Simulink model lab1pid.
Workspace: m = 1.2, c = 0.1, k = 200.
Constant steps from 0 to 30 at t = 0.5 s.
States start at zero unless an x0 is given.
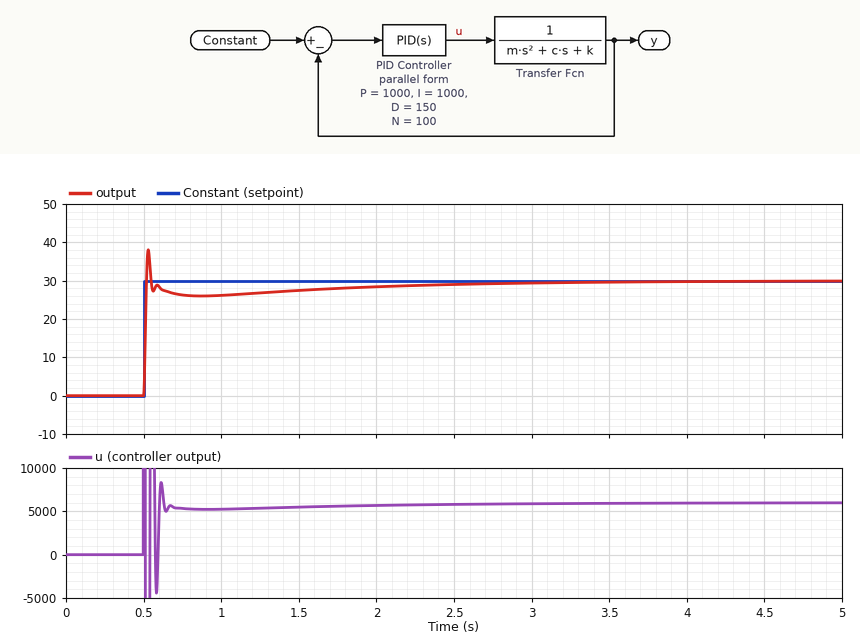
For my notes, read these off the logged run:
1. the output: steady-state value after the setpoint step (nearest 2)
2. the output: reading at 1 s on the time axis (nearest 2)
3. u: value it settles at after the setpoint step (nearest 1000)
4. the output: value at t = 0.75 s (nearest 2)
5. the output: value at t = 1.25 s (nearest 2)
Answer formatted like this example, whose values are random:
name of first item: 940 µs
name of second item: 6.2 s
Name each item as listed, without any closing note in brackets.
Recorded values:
the output: steady-state value after the setpoint step: 30
the output: reading at 1 s on the time axis: 26
u: value it settles at after the setpoint step: 6000
the output: value at t = 0.75 s: 26
the output: value at t = 1.25 s: 26
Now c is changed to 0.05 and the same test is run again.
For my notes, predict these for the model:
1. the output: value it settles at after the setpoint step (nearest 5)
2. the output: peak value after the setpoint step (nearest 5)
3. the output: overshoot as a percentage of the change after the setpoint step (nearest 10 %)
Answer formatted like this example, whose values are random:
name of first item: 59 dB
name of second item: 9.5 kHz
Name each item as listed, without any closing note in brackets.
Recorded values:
the output: value it settles at after the setpoint step: 30
the output: peak value after the setpoint step: 40
the output: overshoot as a percentage of the change after the setpoint step: 30 %
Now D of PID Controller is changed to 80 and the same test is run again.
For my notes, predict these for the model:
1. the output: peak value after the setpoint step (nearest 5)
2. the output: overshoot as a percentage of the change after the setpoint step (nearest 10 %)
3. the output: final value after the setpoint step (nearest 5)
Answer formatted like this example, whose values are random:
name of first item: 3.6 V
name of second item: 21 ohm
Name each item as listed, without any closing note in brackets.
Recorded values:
the output: peak value after the setpoint step: 35
the output: overshoot as a percentage of the change after the setpoint step: 20 %
the output: final value after the setpoint step: 30
